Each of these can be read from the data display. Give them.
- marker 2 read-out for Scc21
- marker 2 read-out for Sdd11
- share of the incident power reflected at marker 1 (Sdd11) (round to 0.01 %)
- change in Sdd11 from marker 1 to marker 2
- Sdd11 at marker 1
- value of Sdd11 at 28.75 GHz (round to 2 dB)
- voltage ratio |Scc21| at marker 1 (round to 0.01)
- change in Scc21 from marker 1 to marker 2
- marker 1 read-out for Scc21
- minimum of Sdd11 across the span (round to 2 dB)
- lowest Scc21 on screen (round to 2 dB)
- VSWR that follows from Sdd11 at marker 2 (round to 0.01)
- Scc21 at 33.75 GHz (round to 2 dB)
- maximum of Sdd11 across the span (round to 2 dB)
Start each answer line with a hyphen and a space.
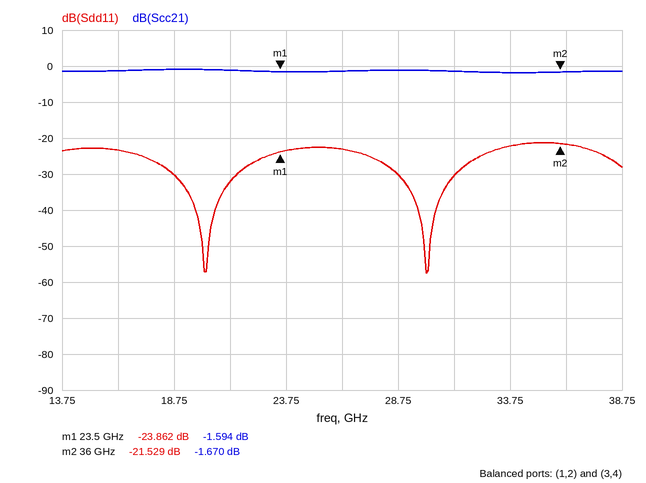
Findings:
- -1.670 dB
- -21.529 dB
- 0.41 %
- 2.333 dB
- -23.862 dB
- -30 dB
- 0.83
- -0.076 dB
- -1.594 dB
- -58 dB
- -2 dB
- 1.18
- -2 dB
- -22 dB
